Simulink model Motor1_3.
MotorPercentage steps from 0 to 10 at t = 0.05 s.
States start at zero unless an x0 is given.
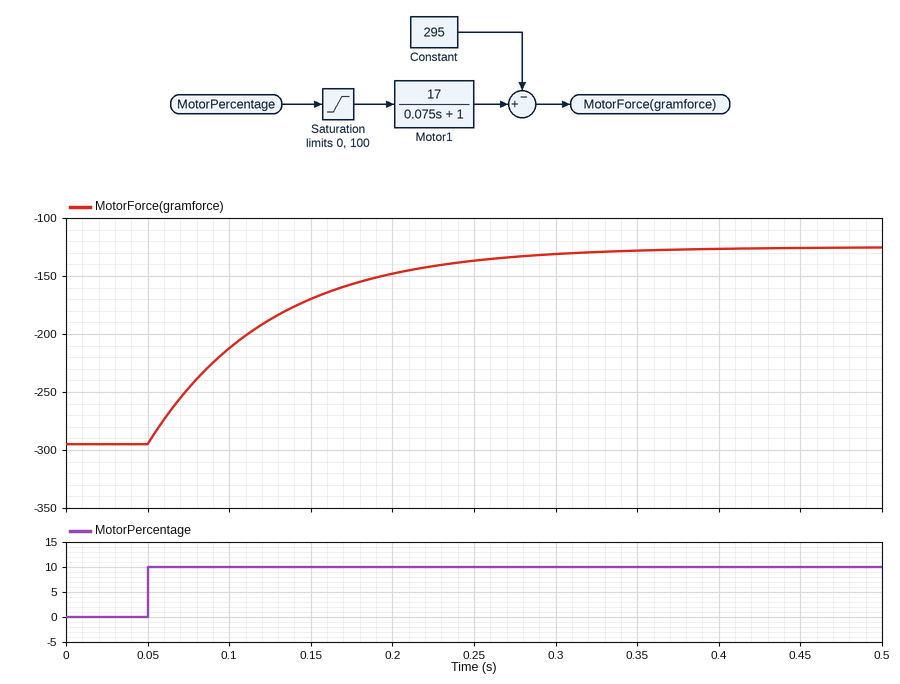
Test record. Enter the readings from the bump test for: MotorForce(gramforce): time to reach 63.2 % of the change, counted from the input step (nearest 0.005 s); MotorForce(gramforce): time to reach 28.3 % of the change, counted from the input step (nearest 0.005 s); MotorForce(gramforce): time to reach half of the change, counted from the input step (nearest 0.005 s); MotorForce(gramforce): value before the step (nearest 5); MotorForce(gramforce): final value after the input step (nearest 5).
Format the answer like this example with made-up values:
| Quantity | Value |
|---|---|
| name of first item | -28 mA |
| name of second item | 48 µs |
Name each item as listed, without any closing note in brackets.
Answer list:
| Quantity | Value |
|---|---|
| MotorForce(gramforce): time to reach 63.2 % of the change, counted from the input step | 0.075 s |
| MotorForce(gramforce): time to reach 28.3 % of the change, counted from the input step | 0.025 s |
| MotorForce(gramforce): time to reach half of the change, counted from the input step | 0.050 s |
| MotorForce(gramforce): value before the step | -295 |
| MotorForce(gramforce): final value after the input step | -125 |
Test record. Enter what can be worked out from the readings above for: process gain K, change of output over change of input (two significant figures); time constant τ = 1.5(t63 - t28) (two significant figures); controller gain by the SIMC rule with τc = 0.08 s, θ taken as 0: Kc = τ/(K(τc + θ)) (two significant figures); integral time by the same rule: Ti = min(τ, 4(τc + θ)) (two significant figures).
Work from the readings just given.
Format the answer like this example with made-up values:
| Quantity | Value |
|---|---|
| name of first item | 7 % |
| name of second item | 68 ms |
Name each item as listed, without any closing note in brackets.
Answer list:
| Quantity | Value |
|---|---|
| process gain K, change of output over change of input | 17 |
| time constant τ = 1.5(t63 - t28) | 0.075 s |
| controller gain by the SIMC rule with τc = 0.08 s, θ taken as 0: Kc = τ/(K(τc + θ)) | 0.055 |
| integral time by the same rule: Ti = min(τ, 4(τc + θ)) | 0.075 s |
